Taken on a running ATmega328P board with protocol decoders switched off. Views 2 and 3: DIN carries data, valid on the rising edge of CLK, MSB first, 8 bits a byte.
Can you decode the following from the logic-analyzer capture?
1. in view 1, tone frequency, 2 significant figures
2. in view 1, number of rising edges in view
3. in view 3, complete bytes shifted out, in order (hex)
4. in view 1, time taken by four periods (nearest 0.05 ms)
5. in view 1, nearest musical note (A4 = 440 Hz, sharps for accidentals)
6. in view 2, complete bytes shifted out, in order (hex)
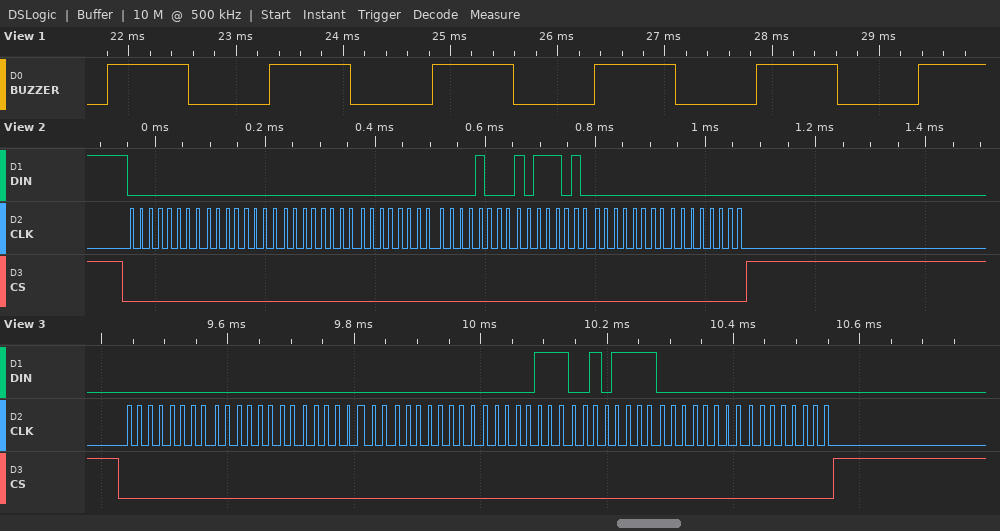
660 Hz
6
0x00 0x00 0x00 0x00 0x07 0x2F 0x00 0x00
6.05 ms
E5
00 00 00 00 08 BA 00 00
